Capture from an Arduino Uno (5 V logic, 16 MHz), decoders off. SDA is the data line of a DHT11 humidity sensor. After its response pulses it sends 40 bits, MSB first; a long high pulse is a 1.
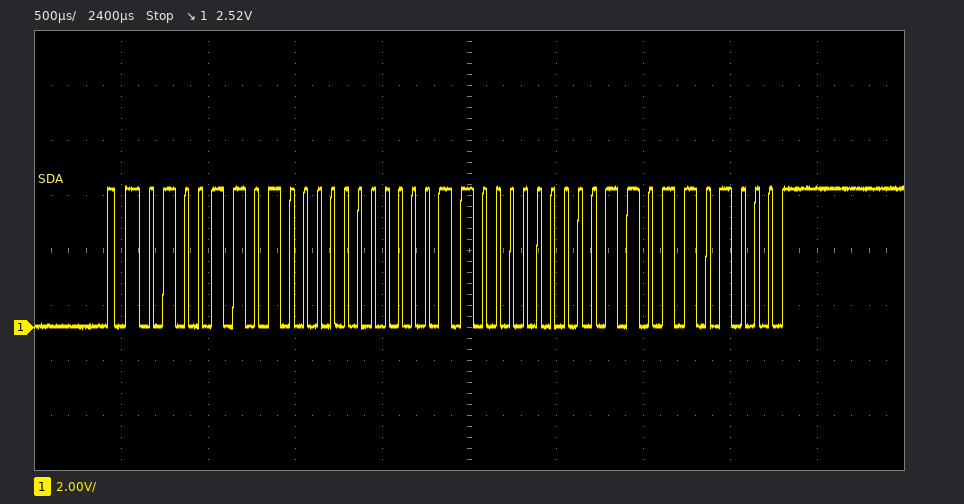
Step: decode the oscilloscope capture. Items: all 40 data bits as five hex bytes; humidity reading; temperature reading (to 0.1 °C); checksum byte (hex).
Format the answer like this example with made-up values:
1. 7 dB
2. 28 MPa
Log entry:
1. 4D 00 18 03 68
2. 77 %
3. 24.3 °C
4. 0x68
